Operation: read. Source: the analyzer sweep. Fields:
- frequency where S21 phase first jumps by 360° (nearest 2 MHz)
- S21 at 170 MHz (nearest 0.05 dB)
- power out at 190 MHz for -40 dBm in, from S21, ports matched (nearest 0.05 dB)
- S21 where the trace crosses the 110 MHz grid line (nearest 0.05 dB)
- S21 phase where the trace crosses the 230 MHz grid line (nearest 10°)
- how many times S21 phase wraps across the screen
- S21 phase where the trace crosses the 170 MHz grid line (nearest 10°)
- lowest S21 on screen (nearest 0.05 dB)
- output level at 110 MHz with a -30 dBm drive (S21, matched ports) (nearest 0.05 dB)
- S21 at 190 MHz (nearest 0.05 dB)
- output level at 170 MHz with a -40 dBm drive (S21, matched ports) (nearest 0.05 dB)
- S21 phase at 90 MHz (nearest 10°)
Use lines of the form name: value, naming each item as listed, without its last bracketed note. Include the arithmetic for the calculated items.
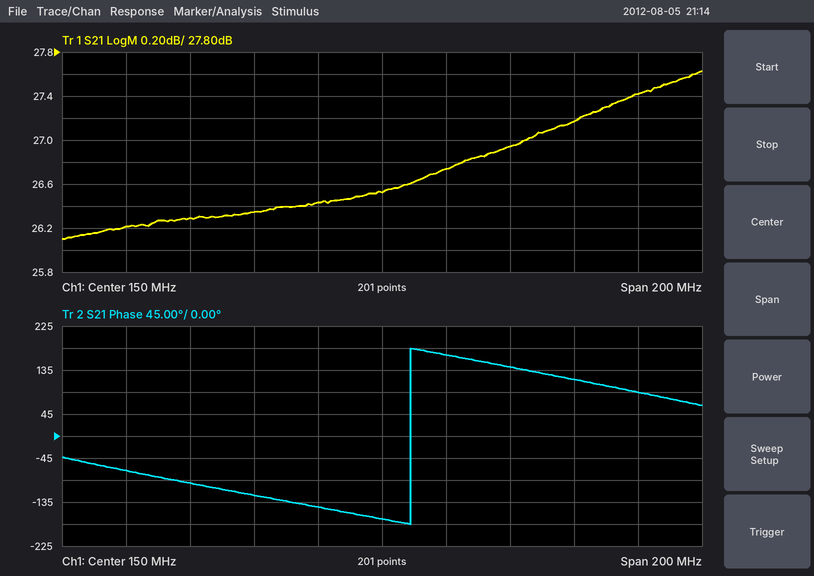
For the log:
frequency where S21 phase first jumps by 360°: 158 MHz
S21 at 170 MHz: 26.75 dB
power out at 190 MHz for -40 dBm in, from S21, ports matched: -40 dBm + (26.95 dB) = -13.05 dBm
S21 where the trace crosses the 110 MHz grid line: 26.35 dB
S21 phase where the trace crosses the 230 MHz grid line: 90°
how many times S21 phase wraps across the screen: 1
S21 phase where the trace crosses the 170 MHz grid line: 170°
lowest S21 on screen: 26.10 dB
output level at 110 MHz with a -30 dBm drive (S21, matched ports): -30 dBm + (26.35 dB) = -3.65 dBm
S21 at 190 MHz: 26.95 dB
output level at 170 MHz with a -40 dBm drive (S21, matched ports): -40 dBm + (26.75 dB) = -13.25 dBm
S21 phase at 90 MHz: -100°
